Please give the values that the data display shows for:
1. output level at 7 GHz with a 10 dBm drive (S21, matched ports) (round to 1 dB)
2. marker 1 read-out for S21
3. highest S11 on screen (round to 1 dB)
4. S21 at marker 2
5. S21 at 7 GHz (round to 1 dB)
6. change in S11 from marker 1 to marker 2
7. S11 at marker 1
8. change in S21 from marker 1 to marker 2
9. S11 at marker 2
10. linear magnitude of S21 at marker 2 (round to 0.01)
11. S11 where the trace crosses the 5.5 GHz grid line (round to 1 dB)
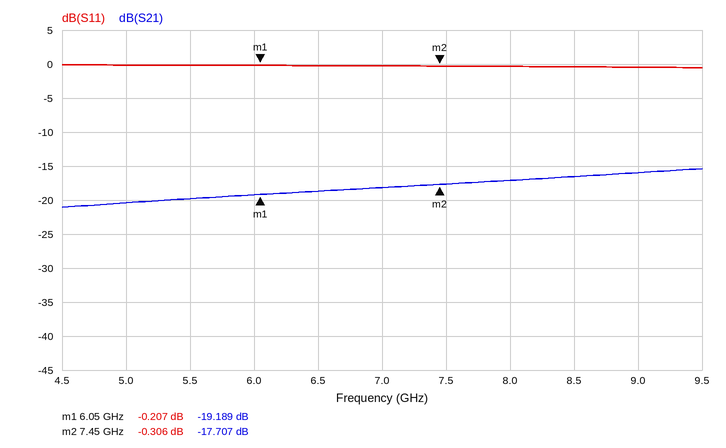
-8 dBm
-19.189 dB
0 dB
-17.707 dB
-18 dB
-0.099 dB
-0.207 dB
1.482 dB
-0.306 dB
0.13
0 dB
